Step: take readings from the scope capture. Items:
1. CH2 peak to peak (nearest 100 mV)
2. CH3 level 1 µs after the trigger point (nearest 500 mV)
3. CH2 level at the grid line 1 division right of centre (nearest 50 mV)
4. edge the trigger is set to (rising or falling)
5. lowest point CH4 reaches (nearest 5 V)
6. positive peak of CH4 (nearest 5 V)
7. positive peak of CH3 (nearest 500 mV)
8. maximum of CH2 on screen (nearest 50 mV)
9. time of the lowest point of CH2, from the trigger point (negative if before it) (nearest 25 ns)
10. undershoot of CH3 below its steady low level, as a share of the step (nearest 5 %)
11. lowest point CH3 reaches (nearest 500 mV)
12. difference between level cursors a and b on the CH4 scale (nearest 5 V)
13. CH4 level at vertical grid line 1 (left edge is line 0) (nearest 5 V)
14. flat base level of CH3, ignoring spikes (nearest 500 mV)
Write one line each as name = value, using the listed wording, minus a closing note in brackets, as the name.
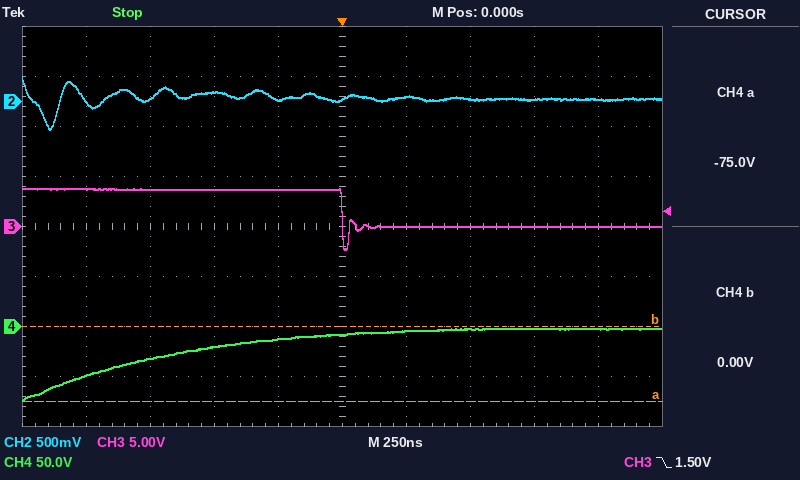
CH2 peak to peak = 500 mV
CH3 level 1 µs after the trigger point = 0.0 V
CH2 level at the grid line 1 division right of centre = 50 mV
edge the trigger is set to = falling
lowest point CH4 reaches = -75 V
positive peak of CH4 = 0 V
positive peak of CH3 = 4.0 V
maximum of CH2 on screen = 250 mV
time of the lowest point of CH2, from the trigger point (negative if before it) = -1.150 µs
undershoot of CH3 below its steady low level, as a share of the step = 60 %
lowest point CH3 reaches = -2.5 V
difference between level cursors a and b on the CH4 scale = 75 V
CH4 level at vertical grid line 1 (left edge is line 0) = -50 V
flat base level of CH3, ignoring spikes = 0.0 V
